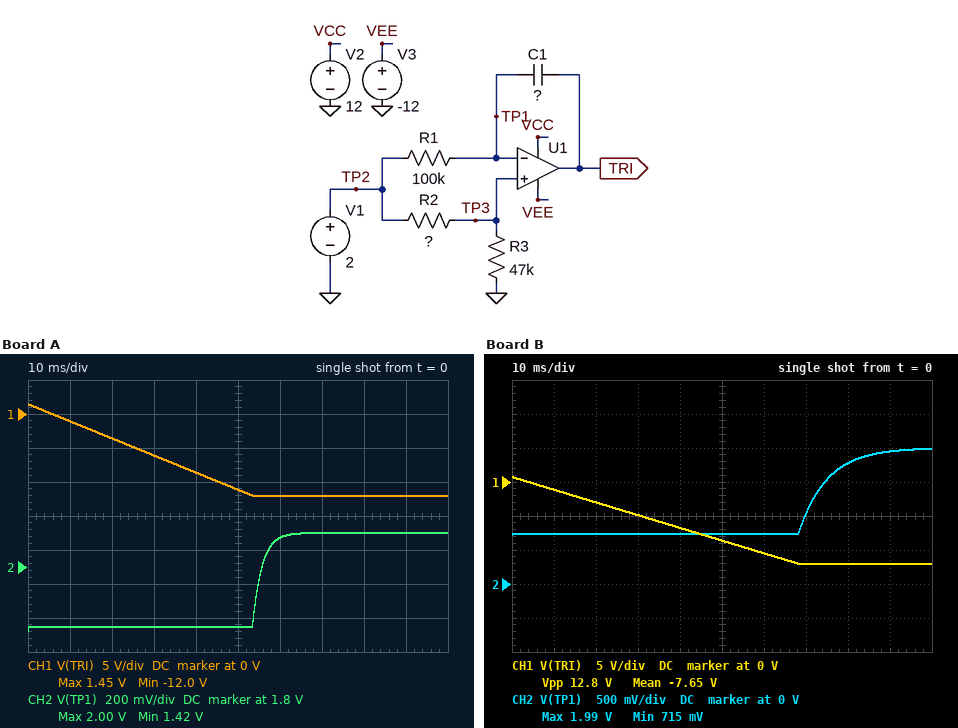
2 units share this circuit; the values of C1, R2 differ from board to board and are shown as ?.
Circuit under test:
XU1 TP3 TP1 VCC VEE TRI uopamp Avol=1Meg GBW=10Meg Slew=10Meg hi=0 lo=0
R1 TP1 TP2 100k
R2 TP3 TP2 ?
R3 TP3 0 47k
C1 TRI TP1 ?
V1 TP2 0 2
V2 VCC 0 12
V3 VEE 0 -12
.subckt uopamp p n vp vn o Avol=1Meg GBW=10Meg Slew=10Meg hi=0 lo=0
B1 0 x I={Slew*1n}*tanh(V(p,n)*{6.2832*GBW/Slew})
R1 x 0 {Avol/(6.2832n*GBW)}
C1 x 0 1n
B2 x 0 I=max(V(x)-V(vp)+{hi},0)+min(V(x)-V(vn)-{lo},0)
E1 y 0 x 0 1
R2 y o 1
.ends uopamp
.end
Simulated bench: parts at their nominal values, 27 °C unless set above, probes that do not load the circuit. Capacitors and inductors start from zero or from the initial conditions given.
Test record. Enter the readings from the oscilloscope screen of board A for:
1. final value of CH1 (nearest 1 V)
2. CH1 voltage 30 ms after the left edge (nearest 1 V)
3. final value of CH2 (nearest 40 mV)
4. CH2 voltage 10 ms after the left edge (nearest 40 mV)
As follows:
-12 V
-6 V
2.00 V
1.44 V
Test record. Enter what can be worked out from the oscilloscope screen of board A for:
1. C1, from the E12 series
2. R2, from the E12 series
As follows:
22 nF
18 kΩ
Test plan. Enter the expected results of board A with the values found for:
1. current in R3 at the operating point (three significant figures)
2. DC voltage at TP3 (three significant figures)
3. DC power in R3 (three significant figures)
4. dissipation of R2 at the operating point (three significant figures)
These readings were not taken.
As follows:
30.8 µA
1.45 V
44.5 µW
17.0 µW
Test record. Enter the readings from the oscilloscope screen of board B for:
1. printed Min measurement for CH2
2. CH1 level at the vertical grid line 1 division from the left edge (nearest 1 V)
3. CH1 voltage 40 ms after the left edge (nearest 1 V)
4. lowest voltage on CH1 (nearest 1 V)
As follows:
715 mV
-1 V
-7 V
-12 V
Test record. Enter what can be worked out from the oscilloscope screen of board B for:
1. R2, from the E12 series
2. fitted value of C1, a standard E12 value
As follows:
82 kΩ
68 nF
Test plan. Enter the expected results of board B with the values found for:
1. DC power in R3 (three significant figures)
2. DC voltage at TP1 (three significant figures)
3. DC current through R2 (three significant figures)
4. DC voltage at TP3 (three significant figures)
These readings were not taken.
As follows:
11.3 µW
2.00 V
15.5 µA
729 mV
